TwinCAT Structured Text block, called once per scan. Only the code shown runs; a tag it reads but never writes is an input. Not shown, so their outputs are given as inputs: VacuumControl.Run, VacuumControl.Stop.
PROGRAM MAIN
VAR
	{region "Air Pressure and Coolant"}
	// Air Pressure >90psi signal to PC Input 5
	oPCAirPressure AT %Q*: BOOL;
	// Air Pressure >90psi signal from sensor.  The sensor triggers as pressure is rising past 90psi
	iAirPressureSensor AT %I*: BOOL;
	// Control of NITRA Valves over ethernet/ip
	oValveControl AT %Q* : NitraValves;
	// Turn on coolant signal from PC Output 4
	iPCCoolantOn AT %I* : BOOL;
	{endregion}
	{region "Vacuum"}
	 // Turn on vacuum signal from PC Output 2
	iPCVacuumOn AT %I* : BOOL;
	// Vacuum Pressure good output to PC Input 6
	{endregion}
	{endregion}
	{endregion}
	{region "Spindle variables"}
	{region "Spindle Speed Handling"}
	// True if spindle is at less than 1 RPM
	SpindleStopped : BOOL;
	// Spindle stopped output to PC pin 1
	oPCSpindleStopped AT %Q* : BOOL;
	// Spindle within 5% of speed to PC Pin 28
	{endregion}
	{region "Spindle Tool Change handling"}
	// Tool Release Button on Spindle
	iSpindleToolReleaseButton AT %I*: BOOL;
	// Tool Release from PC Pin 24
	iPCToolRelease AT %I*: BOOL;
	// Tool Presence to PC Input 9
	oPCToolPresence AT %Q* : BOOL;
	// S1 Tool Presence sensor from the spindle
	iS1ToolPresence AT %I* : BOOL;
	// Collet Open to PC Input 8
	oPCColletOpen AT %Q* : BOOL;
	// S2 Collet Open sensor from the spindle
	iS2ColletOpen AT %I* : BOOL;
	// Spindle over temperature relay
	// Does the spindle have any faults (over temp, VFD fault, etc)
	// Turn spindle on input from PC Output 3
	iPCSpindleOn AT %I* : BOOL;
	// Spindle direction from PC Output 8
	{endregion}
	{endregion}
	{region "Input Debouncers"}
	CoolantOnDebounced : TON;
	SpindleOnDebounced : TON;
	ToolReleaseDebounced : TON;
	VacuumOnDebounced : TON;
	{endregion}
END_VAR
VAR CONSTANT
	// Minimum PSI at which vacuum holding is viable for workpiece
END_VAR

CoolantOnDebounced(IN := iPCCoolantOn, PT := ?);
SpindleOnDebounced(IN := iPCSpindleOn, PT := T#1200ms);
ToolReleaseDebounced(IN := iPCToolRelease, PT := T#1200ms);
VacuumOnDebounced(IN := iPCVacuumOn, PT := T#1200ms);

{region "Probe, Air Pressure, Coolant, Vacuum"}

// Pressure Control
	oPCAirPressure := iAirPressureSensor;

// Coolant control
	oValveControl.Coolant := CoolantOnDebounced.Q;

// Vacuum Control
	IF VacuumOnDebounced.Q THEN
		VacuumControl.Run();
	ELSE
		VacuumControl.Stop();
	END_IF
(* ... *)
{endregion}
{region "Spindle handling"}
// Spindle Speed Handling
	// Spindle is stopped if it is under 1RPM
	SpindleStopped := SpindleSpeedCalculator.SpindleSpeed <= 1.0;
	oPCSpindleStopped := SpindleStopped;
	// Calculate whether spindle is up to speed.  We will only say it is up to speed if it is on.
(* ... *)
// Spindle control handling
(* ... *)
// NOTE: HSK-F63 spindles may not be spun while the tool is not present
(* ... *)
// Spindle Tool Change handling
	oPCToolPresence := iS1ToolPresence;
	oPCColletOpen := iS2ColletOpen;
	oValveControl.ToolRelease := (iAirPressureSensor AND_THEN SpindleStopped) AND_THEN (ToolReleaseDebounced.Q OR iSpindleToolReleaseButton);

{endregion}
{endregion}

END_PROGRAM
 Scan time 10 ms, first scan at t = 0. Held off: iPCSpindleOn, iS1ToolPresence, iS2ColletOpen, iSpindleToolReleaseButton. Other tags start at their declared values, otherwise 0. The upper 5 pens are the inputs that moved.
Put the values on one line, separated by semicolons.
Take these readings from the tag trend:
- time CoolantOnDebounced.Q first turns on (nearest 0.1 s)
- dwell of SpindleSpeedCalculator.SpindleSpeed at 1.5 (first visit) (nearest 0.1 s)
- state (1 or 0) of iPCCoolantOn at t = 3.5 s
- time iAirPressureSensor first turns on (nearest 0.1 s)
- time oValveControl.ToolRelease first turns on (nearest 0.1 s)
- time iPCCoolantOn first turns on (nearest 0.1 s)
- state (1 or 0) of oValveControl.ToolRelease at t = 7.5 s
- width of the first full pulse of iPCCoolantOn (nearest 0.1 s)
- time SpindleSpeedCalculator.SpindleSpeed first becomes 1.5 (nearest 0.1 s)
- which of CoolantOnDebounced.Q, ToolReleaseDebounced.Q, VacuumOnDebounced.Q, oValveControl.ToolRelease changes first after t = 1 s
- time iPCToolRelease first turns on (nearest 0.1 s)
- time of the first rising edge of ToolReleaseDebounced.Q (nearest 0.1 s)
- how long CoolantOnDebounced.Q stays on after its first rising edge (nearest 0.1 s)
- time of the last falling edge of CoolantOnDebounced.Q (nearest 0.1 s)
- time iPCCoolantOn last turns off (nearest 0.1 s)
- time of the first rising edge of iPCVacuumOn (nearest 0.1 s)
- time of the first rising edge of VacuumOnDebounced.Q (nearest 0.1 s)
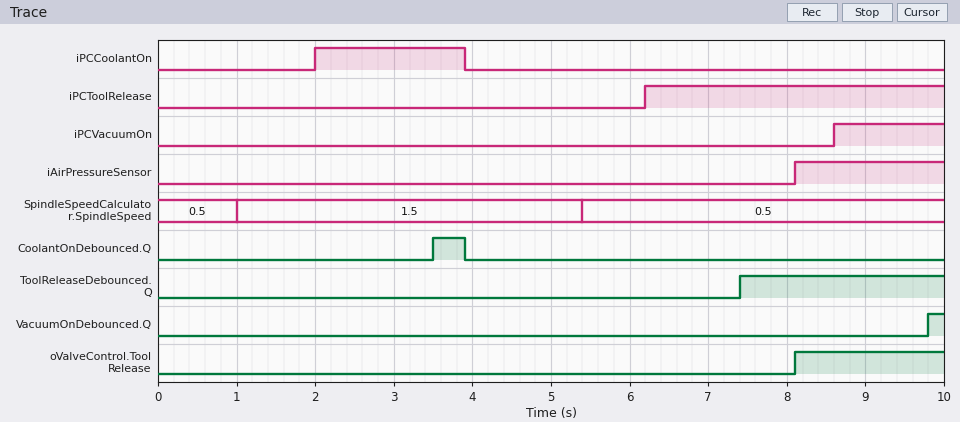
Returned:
3.5 s; 4.4 s; 1; 8.1 s; 8.1 s; 2.0 s; 0; 1.9 s; 1.0 s; CoolantOnDebounced.Q; 6.2 s; 7.4 s; 0.4 s; 3.9 s; 3.9 s; 8.6 s; 9.8 s
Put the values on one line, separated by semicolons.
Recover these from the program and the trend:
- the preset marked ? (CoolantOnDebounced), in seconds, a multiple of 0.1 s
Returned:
1.5 s
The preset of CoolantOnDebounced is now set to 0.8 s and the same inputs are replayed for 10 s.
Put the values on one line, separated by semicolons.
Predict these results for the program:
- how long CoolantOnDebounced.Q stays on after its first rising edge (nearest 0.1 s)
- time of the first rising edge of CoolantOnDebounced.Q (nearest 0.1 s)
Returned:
1.1 s; 2.8 s
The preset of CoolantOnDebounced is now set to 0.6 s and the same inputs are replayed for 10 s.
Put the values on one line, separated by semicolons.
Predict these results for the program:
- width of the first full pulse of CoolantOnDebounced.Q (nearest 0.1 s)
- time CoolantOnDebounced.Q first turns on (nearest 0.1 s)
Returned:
1.3 s; 2.6 s
